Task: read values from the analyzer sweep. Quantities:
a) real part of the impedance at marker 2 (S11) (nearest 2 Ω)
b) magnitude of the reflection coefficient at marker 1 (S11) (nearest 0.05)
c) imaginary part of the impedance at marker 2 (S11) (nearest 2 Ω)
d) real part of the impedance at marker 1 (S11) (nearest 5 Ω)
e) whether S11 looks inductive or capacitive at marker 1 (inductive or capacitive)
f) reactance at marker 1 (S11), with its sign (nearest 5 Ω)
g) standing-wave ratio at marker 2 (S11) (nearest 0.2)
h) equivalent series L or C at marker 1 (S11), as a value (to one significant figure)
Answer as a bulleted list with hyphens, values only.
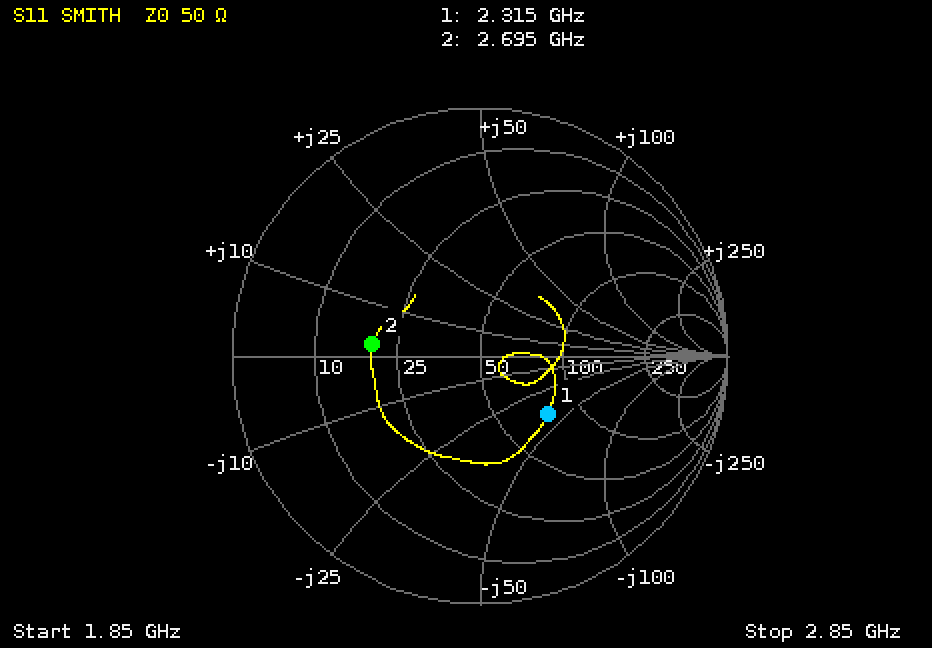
- 20 Ω
- 0.35
- +2 Ω
- 75 Ω
- capacitive
- -40 Ω
- 2.6
- 2 pF
